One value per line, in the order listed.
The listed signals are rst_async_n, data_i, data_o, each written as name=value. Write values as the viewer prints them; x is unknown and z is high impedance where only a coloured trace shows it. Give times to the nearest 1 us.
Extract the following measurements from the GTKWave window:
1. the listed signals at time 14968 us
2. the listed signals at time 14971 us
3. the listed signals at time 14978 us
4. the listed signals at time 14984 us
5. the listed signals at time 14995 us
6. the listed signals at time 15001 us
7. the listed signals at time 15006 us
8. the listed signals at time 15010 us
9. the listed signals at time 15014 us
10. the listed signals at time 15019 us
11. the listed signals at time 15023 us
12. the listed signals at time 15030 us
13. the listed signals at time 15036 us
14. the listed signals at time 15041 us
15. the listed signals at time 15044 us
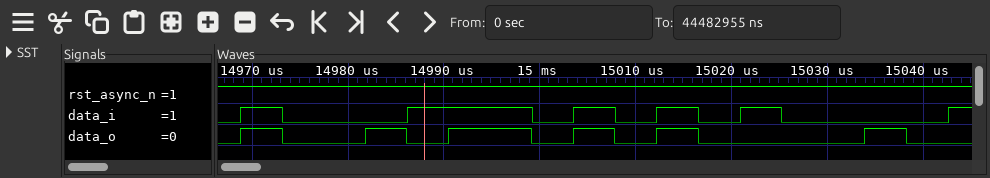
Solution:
rst_async_n=1, data_i=0, data_o=0
rst_async_n=1, data_i=1, data_o=1
rst_async_n=1, data_i=0, data_o=0
rst_async_n=1, data_i=0, data_o=1
rst_async_n=1, data_i=1, data_o=1
rst_async_n=1, data_i=0, data_o=0
rst_async_n=1, data_i=1, data_o=1
rst_async_n=1, data_i=0, data_o=0
rst_async_n=1, data_i=1, data_o=1
rst_async_n=1, data_i=0, data_o=0
rst_async_n=1, data_i=1, data_o=0
rst_async_n=1, data_i=0, data_o=0
rst_async_n=1, data_i=0, data_o=1
rst_async_n=1, data_i=0, data_o=0
rst_async_n=1, data_i=1, data_o=0
